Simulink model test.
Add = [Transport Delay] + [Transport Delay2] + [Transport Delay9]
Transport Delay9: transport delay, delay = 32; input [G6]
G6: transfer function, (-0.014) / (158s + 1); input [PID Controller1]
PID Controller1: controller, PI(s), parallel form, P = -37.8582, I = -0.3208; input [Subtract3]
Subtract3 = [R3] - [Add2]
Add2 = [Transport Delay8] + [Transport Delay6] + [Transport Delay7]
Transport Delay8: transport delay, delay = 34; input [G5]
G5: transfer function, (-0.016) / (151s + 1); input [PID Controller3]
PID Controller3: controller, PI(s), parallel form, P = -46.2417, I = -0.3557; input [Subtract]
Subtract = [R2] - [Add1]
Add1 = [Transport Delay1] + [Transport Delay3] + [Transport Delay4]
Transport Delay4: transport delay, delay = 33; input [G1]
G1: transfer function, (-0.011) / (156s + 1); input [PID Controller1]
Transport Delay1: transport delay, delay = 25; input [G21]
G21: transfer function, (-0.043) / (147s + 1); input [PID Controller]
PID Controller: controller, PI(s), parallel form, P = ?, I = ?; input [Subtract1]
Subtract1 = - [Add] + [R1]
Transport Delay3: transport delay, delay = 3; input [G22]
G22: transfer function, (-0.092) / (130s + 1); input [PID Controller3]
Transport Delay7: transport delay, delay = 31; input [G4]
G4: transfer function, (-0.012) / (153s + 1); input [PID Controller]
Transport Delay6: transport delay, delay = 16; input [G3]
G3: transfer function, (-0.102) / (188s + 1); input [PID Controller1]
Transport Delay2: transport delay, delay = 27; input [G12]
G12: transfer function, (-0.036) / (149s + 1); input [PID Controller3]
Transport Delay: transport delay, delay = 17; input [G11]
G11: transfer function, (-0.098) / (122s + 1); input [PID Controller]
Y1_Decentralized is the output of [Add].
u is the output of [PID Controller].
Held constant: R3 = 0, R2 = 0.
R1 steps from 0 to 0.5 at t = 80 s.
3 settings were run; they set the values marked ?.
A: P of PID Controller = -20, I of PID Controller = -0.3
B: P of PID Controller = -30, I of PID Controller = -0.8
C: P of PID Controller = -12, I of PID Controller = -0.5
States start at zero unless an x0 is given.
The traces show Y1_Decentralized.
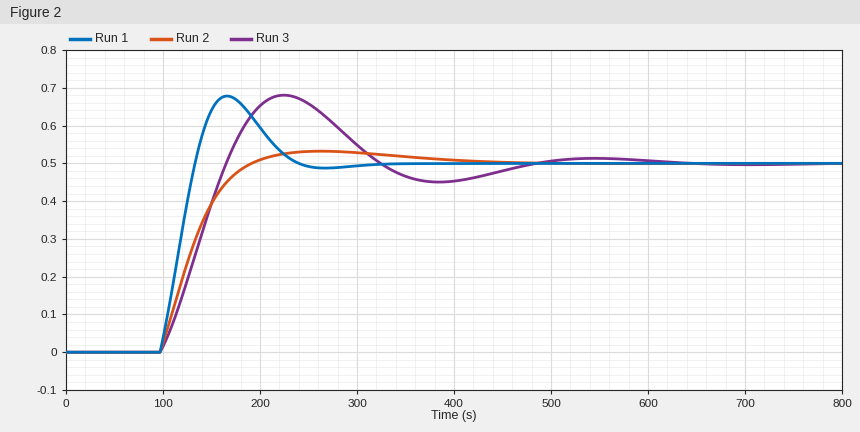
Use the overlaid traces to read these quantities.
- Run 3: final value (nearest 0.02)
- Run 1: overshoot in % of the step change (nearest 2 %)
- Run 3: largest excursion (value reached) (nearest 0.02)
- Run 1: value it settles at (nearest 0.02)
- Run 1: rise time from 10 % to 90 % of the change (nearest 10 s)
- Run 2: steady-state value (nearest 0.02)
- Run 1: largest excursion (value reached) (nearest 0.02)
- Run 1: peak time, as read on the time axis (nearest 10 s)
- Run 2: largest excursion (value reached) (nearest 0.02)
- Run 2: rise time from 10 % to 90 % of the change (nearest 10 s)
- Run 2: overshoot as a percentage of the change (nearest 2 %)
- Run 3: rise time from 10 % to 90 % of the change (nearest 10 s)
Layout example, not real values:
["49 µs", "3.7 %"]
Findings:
["0.50", "36 %", "0.68", "0.50", "30 s", "0.50", "0.68", "170 s", "0.54", "60 s", "6 %", "50 s"]
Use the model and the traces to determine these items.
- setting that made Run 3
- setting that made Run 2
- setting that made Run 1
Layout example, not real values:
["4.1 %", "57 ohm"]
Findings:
["C", "A", "B"]
